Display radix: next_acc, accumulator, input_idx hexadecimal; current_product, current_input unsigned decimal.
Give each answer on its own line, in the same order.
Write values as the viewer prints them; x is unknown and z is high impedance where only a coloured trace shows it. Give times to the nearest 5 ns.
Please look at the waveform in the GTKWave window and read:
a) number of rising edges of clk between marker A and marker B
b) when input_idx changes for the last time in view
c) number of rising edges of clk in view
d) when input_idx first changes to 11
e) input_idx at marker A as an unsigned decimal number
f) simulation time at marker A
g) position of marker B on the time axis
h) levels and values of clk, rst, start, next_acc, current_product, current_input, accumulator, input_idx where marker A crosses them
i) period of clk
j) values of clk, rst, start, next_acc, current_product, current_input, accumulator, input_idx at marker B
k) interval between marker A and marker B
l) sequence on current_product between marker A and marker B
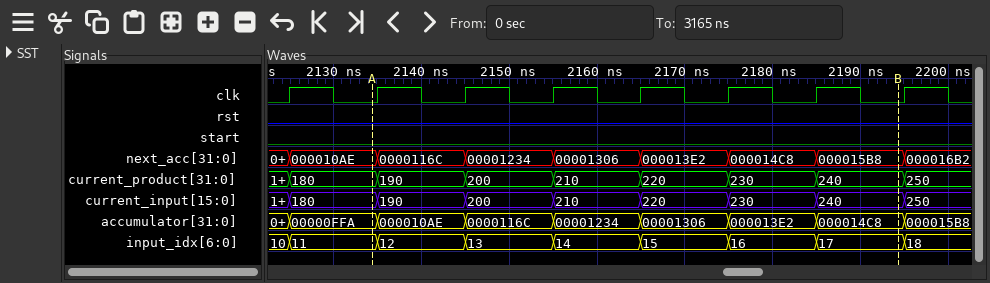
6
2195 ns
8
2125 ns
17
2135 ns
2195 ns
clk=0, rst=0, start=0, next_acc=000010AE, current_product=180, current_input=180, accumulator=00000FFA, input_idx=11
10 ns
clk=0, rst=0, start=0, next_acc=000015B8, current_product=240, current_input=240, accumulator=000014C8, input_idx=17
60 ns
180, 190, 200, 210, 220, 230, 240
